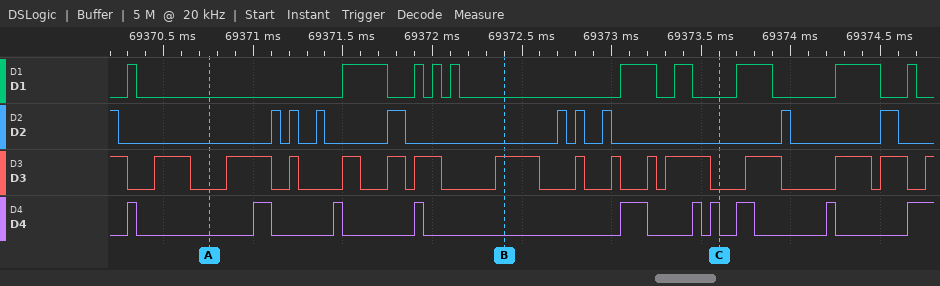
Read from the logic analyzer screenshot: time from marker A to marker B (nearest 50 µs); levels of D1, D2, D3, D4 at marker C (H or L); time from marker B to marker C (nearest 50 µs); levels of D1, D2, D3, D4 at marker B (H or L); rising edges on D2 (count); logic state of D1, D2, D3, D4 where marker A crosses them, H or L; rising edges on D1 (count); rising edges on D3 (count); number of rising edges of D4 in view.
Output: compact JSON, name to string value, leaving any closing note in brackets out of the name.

{"time from marker A to marker B": "1650 µs", "levels of D1, D2, D3, D4 at marker C": "D1=L, D2=L, D3=L, D4=L", "time from marker B to marker C": "1200 µs", "levels of D1, D2, D3, D4 at marker B": "D1=L, D2=L, D3=H, D4=L", "rising edges on D2": "9", "logic state of D1, D2, D3, D4 where marker A crosses them, H or L": "D1=L, D2=L, D3=L, D4=L", "rising edges on D1": "10", "rising edges on D3": "15", "number of rising edges of D4 in view": "10"}
